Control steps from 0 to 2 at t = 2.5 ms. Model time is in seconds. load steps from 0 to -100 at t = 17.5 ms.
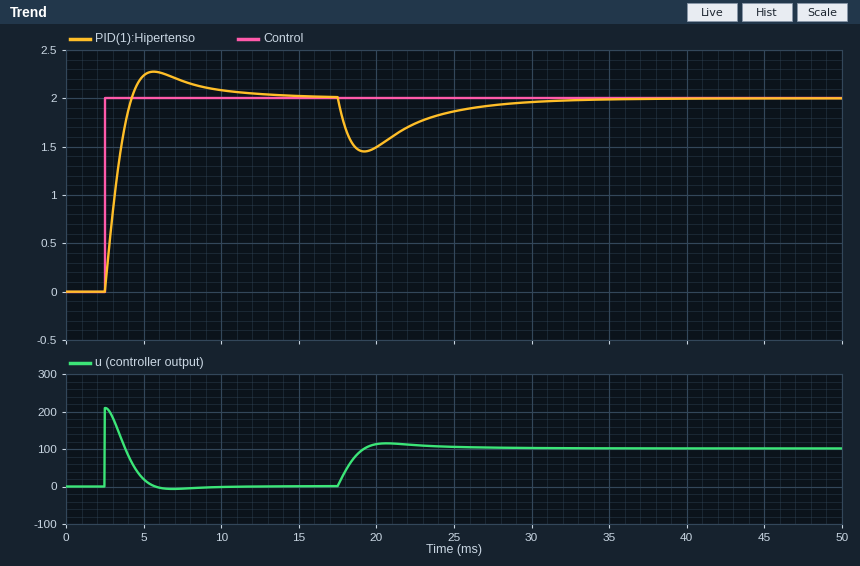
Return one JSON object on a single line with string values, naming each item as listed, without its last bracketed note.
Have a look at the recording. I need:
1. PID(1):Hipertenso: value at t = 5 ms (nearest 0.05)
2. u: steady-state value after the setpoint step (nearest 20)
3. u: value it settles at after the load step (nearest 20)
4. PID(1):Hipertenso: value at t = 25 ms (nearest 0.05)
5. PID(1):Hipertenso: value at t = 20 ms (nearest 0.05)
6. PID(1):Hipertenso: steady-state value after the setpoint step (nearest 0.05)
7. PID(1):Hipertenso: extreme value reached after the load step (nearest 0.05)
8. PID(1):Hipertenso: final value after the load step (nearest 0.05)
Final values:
{"PID(1):Hipertenso: value at t = 5 ms": "2.25", "u: steady-state value after the setpoint step": "0", "u: value it settles at after the load step": "100", "PID(1):Hipertenso: value at t = 25 ms": "1.85", "PID(1):Hipertenso: value at t = 20 ms": "1.50", "PID(1):Hipertenso: steady-state value after the setpoint step": "2.00", "PID(1):Hipertenso: extreme value reached after the load step": "1.45", "PID(1):Hipertenso: final value after the load step": "2.00"}
